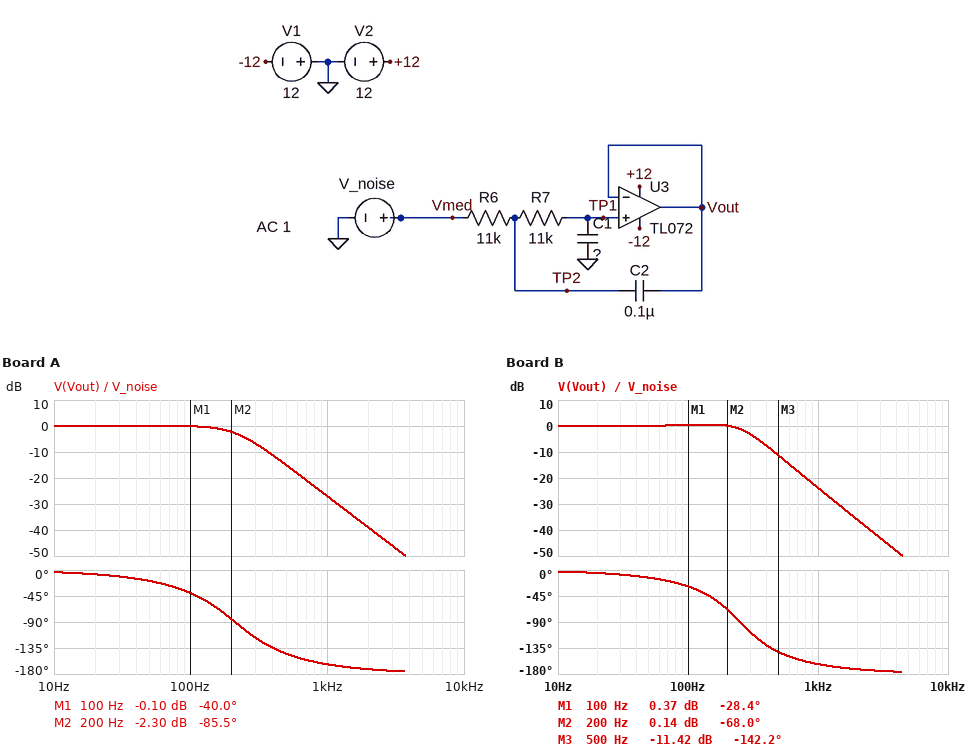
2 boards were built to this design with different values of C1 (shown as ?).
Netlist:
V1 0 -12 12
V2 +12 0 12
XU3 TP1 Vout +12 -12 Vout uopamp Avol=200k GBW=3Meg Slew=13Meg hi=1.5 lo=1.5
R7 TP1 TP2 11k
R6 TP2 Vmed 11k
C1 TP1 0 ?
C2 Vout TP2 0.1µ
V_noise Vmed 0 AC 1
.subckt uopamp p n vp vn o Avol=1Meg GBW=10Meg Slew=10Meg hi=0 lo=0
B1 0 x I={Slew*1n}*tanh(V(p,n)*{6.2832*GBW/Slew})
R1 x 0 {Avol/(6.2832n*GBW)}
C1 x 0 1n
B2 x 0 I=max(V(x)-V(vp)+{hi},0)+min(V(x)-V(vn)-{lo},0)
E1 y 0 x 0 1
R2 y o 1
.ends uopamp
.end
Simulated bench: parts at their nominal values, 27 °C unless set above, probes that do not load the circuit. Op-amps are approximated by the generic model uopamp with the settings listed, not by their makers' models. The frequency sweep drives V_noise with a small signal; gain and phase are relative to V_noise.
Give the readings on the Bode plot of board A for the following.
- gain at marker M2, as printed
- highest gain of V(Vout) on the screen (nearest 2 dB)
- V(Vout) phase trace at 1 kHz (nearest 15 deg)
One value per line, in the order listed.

-2.30 dB
0 dB
-165 deg
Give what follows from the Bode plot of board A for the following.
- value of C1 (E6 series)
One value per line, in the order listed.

47 nF
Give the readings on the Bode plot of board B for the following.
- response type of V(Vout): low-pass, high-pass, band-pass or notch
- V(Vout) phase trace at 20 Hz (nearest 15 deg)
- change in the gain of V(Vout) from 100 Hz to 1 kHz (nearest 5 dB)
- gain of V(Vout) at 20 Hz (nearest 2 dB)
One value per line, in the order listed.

low-pass
0 deg
-25 dB
0 dB
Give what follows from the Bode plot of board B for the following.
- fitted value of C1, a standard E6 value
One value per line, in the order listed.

33 nF
